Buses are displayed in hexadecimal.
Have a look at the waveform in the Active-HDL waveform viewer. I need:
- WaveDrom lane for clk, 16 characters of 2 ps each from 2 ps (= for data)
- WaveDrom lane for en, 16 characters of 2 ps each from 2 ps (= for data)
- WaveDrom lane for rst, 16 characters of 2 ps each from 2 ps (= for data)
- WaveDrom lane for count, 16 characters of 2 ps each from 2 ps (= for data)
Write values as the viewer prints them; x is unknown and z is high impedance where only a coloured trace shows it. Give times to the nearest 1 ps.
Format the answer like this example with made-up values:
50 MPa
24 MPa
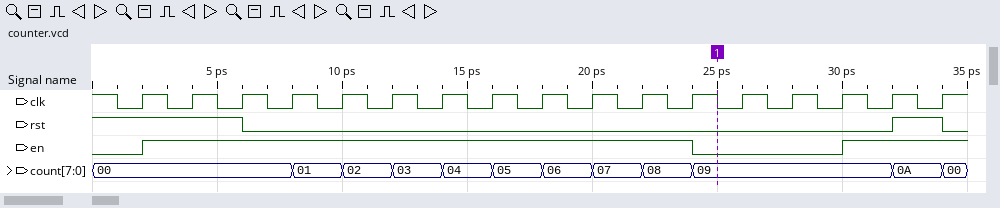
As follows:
{name: 'clk', wave: 'p...............'}
{name: 'en', wave: '1..........0..1.'}
{name: 'rst', wave: '1.0............1'}
{name: 'count', wave: '=..=========...=', data: '00 01 02 03 04 05 06 07 08 09 0A'}
